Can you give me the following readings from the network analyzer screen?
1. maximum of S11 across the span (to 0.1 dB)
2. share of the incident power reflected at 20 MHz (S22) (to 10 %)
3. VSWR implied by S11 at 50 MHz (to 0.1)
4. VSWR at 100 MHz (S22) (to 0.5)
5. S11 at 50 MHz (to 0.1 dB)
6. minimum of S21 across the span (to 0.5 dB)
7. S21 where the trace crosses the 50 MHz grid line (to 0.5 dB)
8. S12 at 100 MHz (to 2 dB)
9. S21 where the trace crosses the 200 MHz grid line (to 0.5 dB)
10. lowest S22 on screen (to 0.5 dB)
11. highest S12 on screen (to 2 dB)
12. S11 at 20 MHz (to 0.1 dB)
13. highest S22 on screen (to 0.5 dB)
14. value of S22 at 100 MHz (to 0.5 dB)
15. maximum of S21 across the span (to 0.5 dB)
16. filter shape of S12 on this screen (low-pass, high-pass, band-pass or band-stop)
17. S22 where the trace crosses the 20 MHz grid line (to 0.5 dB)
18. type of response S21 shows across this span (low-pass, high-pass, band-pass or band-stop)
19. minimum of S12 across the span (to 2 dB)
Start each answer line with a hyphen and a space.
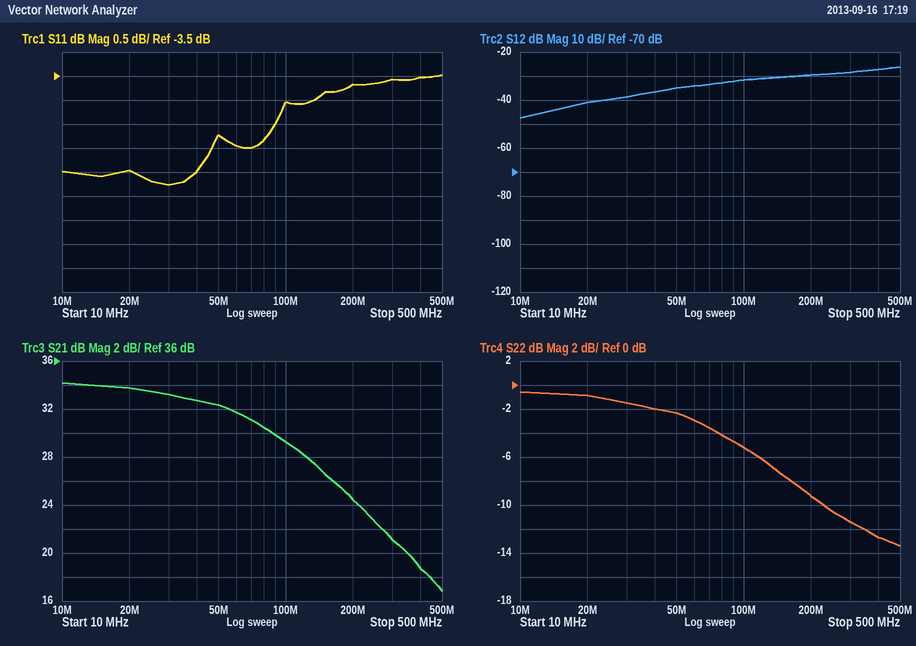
- -3.5 dB
- 80 %
- 3.8
- 3.5
- -4.7 dB
- 17.0 dB
- 32.5 dB
- -32 dB
- 24.5 dB
- -13.5 dB
- -26 dB
- -5.5 dB
- -0.5 dB
- -5.0 dB
- 34.0 dB
- high-pass
- -1.0 dB
- low-pass
- -48 dB
